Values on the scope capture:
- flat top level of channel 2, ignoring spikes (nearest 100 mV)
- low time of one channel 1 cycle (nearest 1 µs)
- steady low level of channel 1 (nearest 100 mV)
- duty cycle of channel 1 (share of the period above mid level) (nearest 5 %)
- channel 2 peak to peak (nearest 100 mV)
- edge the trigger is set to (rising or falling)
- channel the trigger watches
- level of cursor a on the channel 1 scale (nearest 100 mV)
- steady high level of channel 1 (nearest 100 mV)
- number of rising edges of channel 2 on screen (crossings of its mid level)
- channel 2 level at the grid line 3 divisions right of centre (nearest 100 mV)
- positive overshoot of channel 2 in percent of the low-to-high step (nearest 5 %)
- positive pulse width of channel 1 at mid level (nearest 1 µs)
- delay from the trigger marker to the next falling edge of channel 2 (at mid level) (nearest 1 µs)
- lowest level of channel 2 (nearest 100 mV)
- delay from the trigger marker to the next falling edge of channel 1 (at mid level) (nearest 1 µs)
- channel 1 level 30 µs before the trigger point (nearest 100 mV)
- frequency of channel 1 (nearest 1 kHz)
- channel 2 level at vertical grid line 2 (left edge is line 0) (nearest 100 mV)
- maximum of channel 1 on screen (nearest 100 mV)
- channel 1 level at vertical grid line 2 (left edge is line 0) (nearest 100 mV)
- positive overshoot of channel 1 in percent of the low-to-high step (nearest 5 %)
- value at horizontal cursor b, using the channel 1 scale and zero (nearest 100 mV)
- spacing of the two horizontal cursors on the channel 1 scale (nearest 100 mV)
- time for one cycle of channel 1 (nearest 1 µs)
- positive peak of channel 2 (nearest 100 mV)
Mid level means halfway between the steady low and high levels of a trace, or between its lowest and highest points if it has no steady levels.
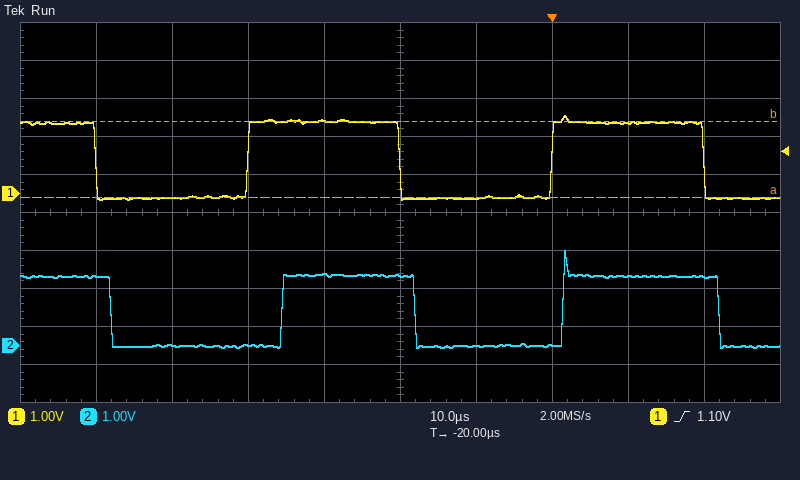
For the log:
1.8 V
20 µs
-100 mV
50 %
2.6 V
rising
channel 1
-100 mV
1.9 V
2
1.8 V
35 %
20 µs
22 µs
-100 mV
20 µs
1.9 V
25 kHz
0.0 V
2.1 V
-100 mV
10 %
1.9 V
2.0 V
40 µs
2.5 V
